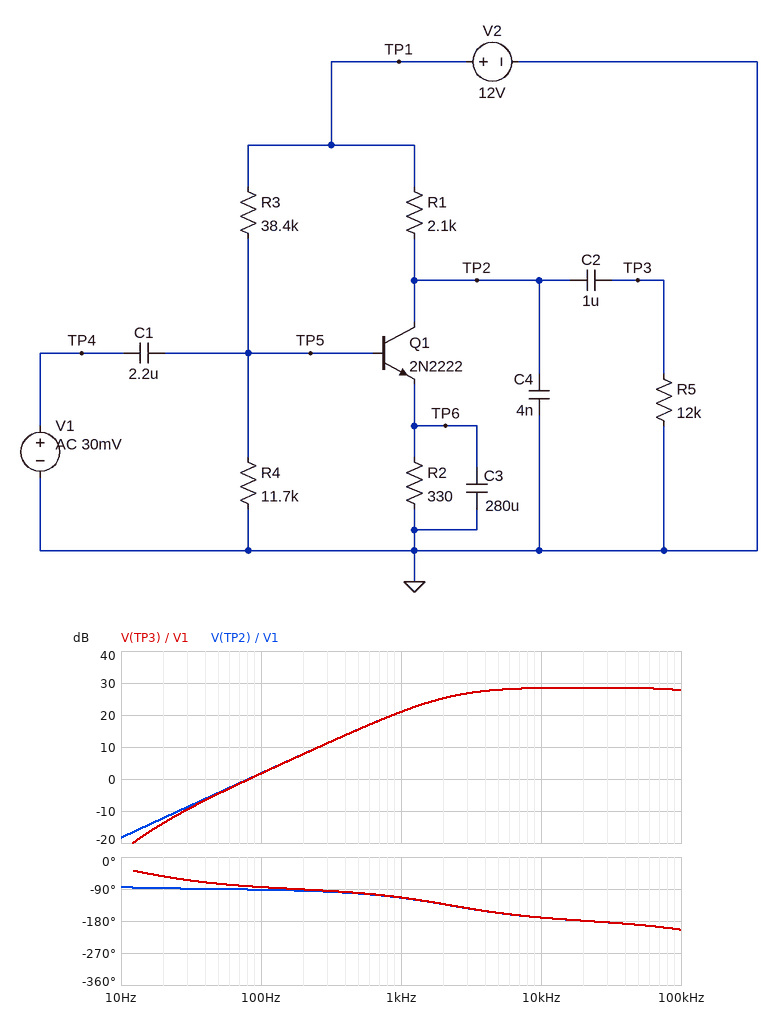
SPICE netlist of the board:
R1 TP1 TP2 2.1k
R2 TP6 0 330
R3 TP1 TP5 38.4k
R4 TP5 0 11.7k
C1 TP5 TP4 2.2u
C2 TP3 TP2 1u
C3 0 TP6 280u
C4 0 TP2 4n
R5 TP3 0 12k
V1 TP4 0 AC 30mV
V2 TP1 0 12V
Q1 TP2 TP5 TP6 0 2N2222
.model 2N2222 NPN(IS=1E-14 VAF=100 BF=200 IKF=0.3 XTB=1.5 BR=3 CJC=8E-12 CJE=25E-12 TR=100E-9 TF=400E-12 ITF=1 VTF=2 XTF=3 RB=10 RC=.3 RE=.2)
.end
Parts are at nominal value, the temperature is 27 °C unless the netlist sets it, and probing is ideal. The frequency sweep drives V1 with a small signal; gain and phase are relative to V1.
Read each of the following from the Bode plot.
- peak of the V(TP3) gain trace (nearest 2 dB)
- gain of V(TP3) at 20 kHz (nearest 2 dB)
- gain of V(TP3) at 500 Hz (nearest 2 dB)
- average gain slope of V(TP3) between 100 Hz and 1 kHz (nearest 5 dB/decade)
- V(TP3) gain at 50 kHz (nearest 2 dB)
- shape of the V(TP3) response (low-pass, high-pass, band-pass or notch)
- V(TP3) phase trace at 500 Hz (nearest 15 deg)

28 dB
28 dB
16 dB
20 dB/decade
28 dB
high-pass
-105 deg
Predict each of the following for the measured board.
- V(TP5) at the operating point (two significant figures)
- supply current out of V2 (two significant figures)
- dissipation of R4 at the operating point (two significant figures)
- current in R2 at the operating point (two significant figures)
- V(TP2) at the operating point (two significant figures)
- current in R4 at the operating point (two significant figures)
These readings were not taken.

2.3 V
5.1 mA
460 µW
4.9 mA
1.7 V
200 µA
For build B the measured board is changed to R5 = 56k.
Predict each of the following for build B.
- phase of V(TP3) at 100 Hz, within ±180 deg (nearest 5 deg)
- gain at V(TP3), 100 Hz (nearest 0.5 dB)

-90 deg
2.0 dB
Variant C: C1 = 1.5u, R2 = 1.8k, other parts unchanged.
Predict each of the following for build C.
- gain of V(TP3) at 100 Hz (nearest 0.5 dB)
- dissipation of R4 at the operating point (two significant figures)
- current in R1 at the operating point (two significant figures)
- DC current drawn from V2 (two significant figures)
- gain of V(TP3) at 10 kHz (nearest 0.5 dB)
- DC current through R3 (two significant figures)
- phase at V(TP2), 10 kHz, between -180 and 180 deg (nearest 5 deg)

36.5 dB
650 µW
1.2 mA
1.4 mA
37.0 dB
240 µA
155 deg
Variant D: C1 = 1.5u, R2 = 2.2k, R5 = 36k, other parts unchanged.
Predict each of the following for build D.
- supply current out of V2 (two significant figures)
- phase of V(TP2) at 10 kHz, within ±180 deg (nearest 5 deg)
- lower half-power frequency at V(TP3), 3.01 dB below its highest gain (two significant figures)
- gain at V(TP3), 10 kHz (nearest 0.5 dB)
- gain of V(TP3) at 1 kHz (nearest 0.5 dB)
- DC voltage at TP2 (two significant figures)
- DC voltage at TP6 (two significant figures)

1.2 mA
155 deg
46 Hz
36.0 dB
37.0 dB
10 V
2.1 V
